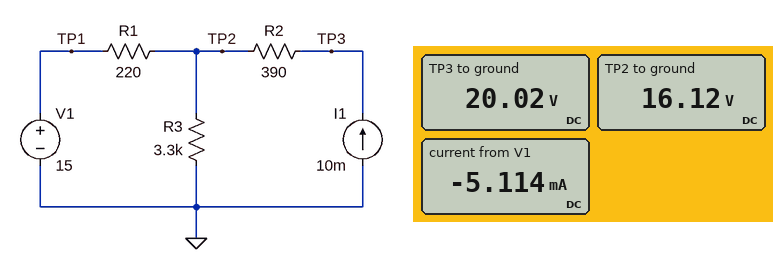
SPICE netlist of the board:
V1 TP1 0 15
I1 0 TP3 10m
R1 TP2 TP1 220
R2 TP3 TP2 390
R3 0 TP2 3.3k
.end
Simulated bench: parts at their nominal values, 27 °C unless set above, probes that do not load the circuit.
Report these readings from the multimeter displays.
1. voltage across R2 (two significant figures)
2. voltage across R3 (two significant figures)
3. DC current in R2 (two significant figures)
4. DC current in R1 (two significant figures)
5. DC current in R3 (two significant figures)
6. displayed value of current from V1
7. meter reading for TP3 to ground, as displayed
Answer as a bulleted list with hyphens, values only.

- 3.9 V
- 16 V
- 10 mA
- 5.1 mA
- 4.9 mA
- -5.114 mA
- 20.02 V
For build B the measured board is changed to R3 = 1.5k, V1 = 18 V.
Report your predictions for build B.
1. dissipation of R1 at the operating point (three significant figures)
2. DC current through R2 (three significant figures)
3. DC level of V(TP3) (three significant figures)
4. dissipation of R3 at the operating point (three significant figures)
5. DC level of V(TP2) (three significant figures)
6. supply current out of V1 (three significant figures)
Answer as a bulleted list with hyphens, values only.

- 669 µW
- 10.0 mA
- 21.5 V
- 207 mW
- 17.6 V
- 1.74 mA
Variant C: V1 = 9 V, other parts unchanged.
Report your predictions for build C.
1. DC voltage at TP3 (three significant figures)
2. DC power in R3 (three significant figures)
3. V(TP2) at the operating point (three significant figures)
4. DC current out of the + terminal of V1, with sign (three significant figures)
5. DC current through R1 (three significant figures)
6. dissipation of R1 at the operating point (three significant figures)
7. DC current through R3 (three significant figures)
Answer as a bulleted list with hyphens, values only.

- 14.4 V
- 33.4 mW
- 10.5 V
- -6.82 mA
- 6.82 mA
- 10.2 mW
- 3.18 mA
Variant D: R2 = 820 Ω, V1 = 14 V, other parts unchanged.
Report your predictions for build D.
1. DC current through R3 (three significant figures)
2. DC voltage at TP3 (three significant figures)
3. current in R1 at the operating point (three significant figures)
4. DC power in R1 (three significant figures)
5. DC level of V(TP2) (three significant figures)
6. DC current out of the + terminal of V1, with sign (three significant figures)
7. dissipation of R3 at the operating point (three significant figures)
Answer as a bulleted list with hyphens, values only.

- 4.60 mA
- 23.4 V
- 5.40 mA
- 6.41 mW
- 15.2 V
- -5.40 mA
- 69.9 mW
